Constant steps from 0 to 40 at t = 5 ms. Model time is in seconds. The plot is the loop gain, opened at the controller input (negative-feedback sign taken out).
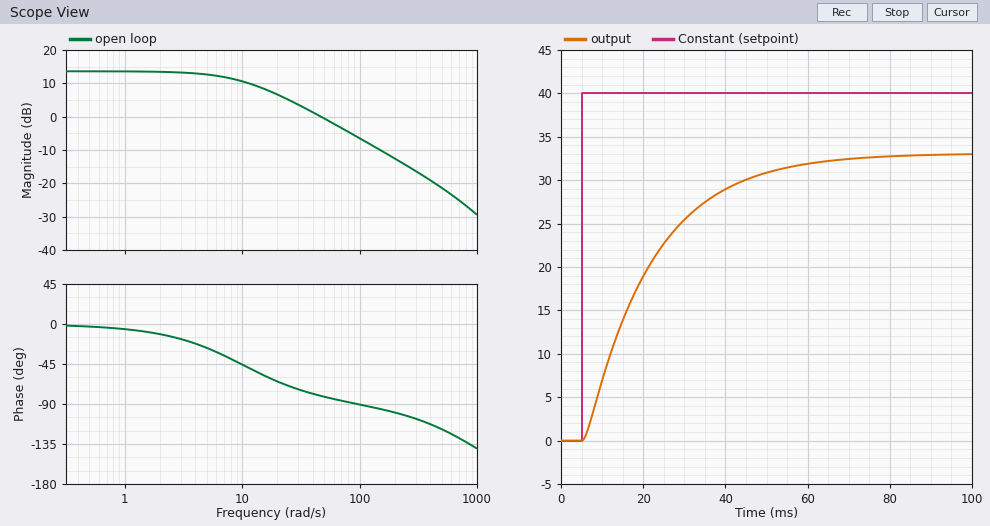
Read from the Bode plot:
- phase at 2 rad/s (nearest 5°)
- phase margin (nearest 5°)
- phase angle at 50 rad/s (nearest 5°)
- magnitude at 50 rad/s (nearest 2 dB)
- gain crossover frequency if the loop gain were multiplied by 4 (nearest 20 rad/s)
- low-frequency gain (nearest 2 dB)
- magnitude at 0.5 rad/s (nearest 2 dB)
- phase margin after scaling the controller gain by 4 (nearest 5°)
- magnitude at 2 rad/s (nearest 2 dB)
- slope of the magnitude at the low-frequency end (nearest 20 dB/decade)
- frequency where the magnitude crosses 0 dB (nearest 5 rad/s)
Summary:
-10°
100°
-80°
0 dB
180 rad/s
14 dB
14 dB
80°
14 dB
0 dB/decade
45 rad/s
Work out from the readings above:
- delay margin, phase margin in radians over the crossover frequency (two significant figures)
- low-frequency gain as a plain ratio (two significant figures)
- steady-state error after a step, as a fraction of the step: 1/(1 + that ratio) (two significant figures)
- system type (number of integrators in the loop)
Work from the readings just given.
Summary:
0.039 s
5.0
0.17
0
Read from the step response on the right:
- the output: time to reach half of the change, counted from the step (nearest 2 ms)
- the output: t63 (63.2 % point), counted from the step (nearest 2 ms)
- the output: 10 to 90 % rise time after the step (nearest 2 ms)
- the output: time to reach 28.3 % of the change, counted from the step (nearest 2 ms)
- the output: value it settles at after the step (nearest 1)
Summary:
12 ms
18 ms
36 ms
6 ms
33
